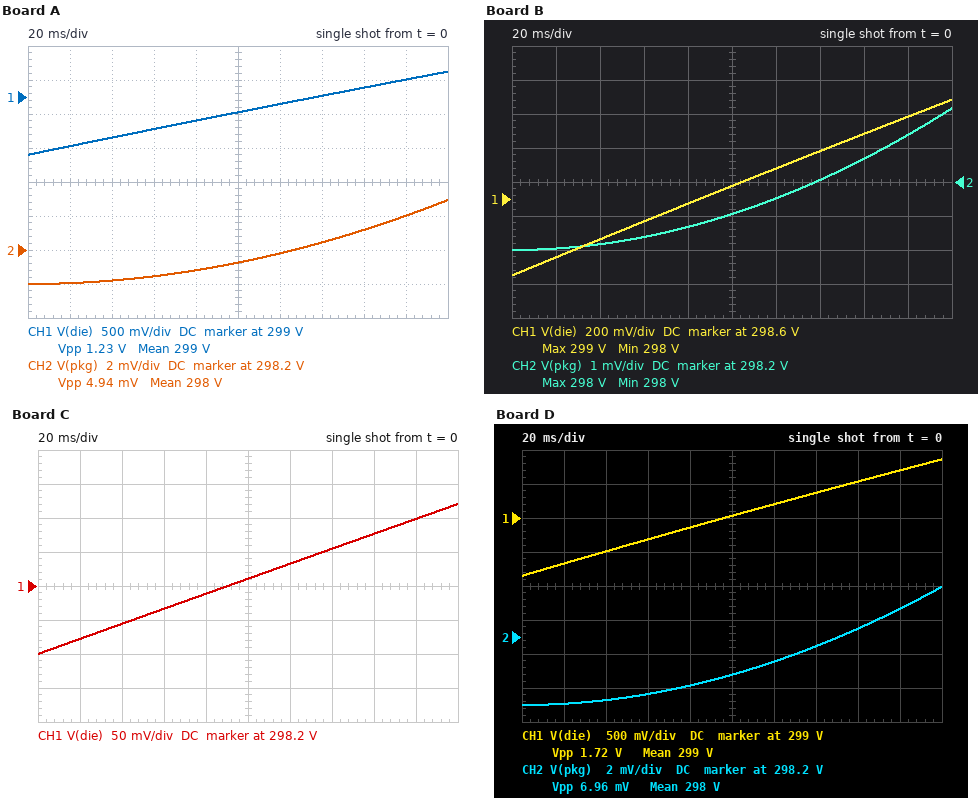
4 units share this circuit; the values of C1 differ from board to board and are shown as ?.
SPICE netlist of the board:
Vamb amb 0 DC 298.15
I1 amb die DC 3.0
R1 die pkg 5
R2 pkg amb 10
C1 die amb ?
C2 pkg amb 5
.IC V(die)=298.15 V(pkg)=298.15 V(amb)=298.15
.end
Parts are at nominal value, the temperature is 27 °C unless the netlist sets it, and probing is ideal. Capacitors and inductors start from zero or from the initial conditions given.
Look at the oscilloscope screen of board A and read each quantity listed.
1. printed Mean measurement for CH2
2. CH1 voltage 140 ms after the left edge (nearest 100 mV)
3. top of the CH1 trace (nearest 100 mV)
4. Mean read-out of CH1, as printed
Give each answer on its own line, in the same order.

298 V
299.0 V
299.4 V
299 V
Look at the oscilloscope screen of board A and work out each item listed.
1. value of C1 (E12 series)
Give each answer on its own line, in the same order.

470 mF
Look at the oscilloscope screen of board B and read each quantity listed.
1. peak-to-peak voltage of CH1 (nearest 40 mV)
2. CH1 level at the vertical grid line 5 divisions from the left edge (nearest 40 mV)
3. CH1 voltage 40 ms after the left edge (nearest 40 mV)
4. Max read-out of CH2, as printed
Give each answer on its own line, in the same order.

1.04 V
298.68 V
298.36 V
298 V
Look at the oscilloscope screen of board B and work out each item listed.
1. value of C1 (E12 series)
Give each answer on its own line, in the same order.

560 mF
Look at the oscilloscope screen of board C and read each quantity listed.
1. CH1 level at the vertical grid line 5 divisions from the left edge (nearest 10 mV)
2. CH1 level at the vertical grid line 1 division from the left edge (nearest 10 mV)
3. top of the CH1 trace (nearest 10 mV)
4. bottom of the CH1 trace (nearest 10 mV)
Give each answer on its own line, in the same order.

298.26 V
298.17 V
298.37 V
298.15 V
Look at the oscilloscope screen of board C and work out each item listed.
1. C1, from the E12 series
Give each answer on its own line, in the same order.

2.7 F
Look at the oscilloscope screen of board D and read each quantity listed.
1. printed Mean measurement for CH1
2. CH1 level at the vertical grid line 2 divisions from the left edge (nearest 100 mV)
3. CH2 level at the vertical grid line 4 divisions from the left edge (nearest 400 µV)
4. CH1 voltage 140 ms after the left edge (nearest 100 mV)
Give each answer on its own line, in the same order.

299 V
298.5 V
298.1512 V
299.4 V
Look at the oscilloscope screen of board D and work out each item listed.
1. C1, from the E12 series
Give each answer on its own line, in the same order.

330 mF
